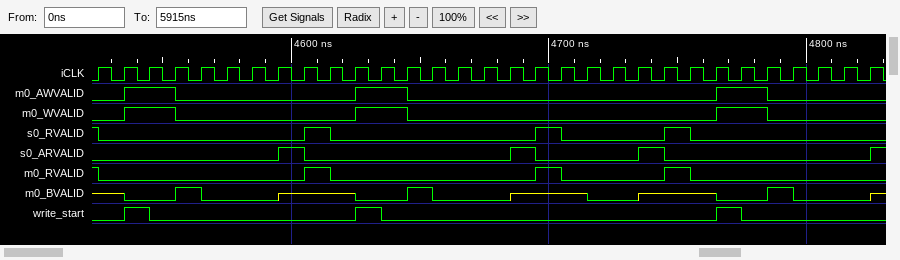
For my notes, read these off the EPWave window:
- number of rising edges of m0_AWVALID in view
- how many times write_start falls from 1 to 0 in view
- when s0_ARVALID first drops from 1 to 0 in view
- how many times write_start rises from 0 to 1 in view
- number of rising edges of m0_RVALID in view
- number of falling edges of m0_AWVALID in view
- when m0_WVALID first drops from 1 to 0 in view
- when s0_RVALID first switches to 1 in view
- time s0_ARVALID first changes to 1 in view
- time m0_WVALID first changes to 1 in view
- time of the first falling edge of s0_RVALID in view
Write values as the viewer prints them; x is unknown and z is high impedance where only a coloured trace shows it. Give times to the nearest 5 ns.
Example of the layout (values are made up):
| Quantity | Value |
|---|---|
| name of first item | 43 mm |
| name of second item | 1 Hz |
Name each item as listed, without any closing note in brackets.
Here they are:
| Quantity | Value |
|---|---|
| number of rising edges of m0_AWVALID in view | 3 |
| how many times write_start falls from 1 to 0 in view | 3 |
| when s0_ARVALID first drops from 1 to 0 in view | 4605 ns |
| how many times write_start rises from 0 to 1 in view | 3 |
| number of rising edges of m0_RVALID in view | 3 |
| number of falling edges of m0_AWVALID in view | 3 |
| when m0_WVALID first drops from 1 to 0 in view | 4555 ns |
| when s0_RVALID first switches to 1 in view | 4605 ns |
| time s0_ARVALID first changes to 1 in view | 4595 ns |
| time m0_WVALID first changes to 1 in view | 4535 ns |
| time of the first falling edge of s0_RVALID in view | 4525 ns |
